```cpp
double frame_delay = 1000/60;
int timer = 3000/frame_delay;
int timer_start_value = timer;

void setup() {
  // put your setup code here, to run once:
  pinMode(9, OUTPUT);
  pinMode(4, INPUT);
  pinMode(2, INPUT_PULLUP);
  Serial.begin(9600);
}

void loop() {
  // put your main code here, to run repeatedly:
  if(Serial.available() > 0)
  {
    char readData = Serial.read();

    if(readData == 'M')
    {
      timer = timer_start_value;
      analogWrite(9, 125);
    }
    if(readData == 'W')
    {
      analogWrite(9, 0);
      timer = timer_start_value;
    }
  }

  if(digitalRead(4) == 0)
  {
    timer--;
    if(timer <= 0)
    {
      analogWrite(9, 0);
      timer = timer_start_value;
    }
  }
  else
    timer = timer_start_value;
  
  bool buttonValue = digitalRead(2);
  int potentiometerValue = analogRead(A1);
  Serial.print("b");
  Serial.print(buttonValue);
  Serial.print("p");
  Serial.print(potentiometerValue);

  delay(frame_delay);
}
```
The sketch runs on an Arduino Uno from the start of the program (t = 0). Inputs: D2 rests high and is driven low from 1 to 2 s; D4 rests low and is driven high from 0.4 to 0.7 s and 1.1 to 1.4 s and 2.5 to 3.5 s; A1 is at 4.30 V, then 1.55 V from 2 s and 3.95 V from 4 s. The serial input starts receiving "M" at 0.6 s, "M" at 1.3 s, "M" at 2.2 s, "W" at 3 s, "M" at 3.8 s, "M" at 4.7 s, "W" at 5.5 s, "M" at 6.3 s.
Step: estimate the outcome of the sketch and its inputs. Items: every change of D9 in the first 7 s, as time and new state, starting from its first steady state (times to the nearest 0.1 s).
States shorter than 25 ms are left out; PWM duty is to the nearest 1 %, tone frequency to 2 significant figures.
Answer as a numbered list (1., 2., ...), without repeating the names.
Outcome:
1. 0 s low; 0.6 s PWM 49 %; 3 s low; 3.8 s PWM 49 %; 5.5 s low; 6.3 s PWM 49 %
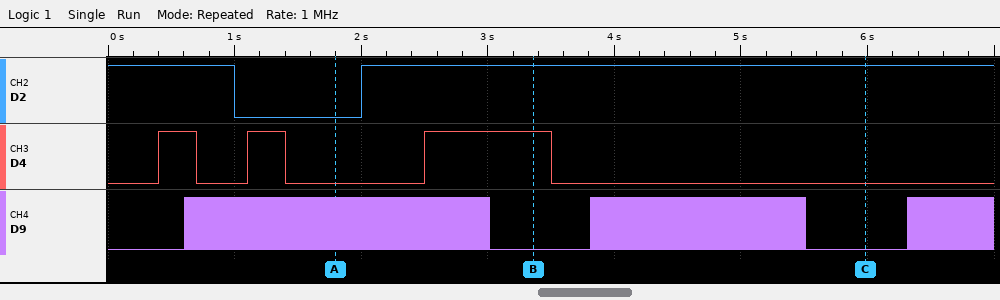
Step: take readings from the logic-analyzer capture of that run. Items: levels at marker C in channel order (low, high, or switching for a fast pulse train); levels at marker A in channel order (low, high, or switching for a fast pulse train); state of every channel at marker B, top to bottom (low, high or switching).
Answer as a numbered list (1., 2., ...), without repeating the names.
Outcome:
1. D2 high, D4 low, D9 low
2. D2 low, D4 low, D9 switching
3. D2 high, D4 high, D9 low
